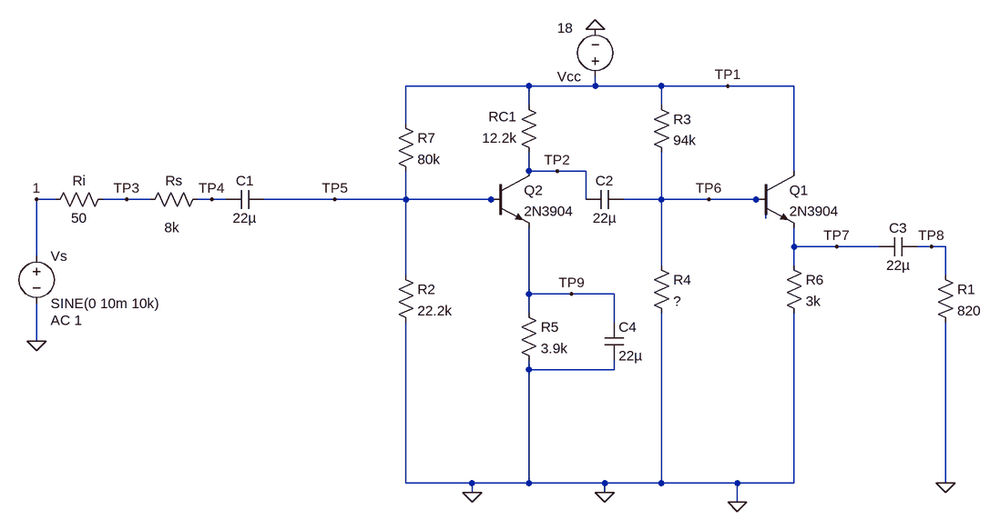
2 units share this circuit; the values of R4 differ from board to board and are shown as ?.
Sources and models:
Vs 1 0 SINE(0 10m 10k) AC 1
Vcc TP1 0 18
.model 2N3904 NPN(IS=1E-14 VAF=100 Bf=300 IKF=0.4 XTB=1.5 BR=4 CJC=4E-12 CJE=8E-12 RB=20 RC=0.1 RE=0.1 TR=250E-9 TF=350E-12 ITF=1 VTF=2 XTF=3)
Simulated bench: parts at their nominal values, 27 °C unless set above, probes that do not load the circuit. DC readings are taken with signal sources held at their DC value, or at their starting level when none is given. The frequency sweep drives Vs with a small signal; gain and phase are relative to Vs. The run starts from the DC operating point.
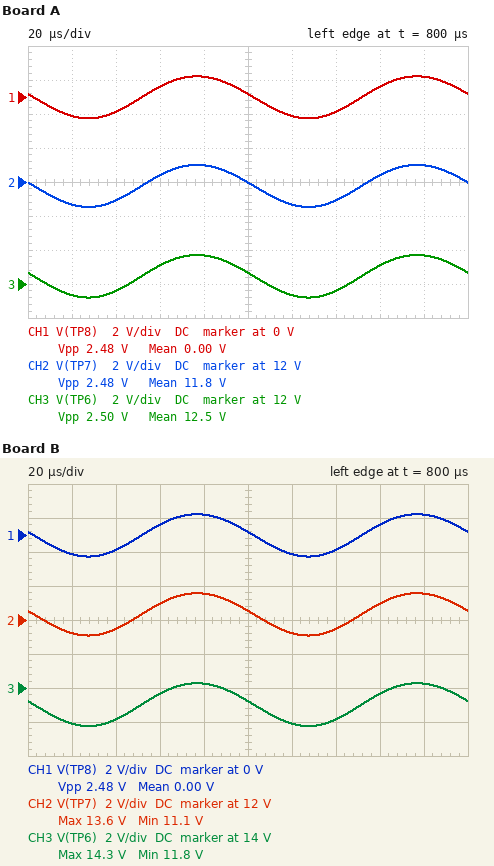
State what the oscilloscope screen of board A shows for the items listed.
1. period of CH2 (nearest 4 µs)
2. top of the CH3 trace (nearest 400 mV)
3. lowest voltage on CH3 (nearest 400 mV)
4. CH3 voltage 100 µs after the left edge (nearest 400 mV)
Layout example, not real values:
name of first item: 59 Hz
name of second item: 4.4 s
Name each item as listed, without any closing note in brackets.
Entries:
period of CH2: 100 µs
top of the CH3 trace: 13.6 V
lowest voltage on CH3: 11.2 V
CH3 voltage 100 µs after the left edge: 12.8 V
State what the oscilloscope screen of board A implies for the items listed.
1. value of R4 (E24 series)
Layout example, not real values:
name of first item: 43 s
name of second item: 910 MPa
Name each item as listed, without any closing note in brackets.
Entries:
value of R4: 270 kΩ
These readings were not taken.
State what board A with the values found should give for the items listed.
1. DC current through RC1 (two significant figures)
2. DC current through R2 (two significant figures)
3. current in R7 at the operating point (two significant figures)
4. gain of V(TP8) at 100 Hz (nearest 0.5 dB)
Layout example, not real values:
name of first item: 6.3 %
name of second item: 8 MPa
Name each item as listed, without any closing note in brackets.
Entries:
DC current through RC1: 820 µA
DC current through R2: 170 µA
current in R7 at the operating point: 180 µA
gain of V(TP8) at 100 Hz: 37.5 dB
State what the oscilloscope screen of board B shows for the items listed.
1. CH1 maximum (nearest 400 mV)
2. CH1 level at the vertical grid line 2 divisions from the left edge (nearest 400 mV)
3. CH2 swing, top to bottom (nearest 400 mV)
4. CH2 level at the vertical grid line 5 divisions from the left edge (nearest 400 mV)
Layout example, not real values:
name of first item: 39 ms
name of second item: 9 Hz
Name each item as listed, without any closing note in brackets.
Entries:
CH1 maximum: 1.2 V
CH1 level at the vertical grid line 2 divisions from the left edge: -800 mV
CH2 swing, top to bottom: 2.4 V
CH2 level at the vertical grid line 5 divisions from the left edge: 12.4 V
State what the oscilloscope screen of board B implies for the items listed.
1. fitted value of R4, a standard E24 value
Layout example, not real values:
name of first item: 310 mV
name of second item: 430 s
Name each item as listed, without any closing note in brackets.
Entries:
fitted value of R4, a standard E24 value: 330 kΩ
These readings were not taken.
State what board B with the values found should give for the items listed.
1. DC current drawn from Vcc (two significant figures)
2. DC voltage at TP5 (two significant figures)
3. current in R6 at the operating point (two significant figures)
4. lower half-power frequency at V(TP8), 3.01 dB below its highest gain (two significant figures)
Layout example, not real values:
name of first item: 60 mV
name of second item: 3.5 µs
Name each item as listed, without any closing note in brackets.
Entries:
DC current drawn from Vcc: 5.2 mA
DC voltage at TP5: 3.9 V
current in R6 at the operating point: 4.1 mA
lower half-power frequency at V(TP8), 3.01 dB below its highest gain: 140 Hz
